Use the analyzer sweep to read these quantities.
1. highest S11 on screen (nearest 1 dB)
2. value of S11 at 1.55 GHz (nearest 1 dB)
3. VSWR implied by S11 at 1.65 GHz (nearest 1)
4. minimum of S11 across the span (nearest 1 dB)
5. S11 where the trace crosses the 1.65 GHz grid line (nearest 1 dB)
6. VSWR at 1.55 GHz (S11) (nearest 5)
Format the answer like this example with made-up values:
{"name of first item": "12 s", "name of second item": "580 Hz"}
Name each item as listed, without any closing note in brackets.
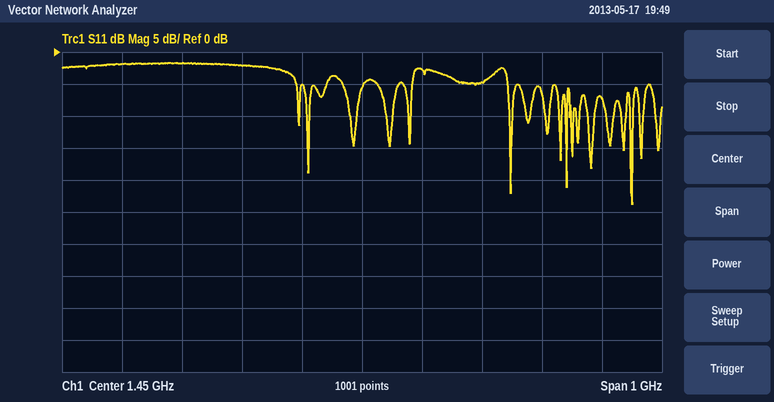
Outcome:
{"highest S11 on screen": "-2 dB", "value of S11 at 1.55 GHz": "-3 dB", "VSWR implied by S11 at 1.65 GHz": "4", "minimum of S11 across the span": "-24 dB", "S11 where the trace crosses the 1.65 GHz grid line": "-5 dB", "VSWR at 1.55 GHz (S11)": "5"}
